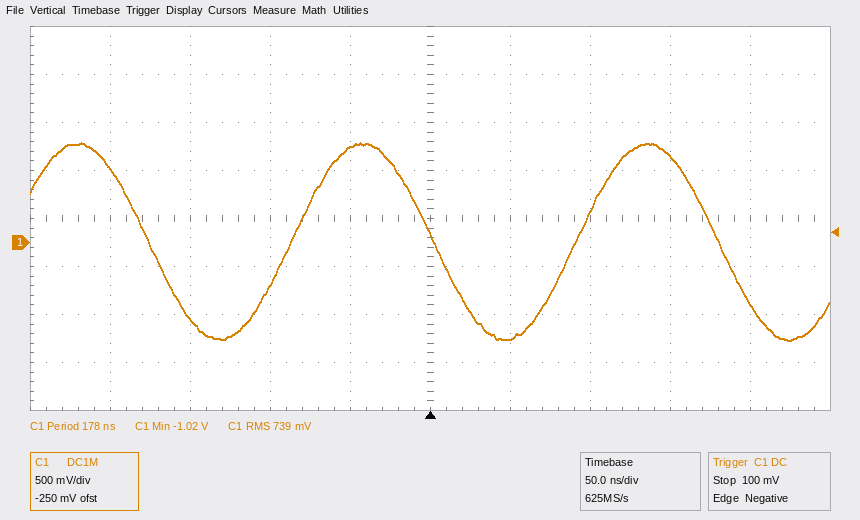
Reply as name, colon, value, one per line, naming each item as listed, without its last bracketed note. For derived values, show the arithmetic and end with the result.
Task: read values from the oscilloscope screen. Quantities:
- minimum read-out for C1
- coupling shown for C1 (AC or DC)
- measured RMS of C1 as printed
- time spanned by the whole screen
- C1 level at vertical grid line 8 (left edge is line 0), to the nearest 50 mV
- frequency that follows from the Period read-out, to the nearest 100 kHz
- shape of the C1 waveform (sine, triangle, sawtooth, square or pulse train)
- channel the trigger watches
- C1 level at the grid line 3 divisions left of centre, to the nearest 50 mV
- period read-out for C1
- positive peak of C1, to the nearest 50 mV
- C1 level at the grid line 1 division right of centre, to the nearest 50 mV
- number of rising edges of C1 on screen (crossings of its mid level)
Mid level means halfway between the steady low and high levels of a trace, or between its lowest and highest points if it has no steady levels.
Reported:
minimum read-out for C1: -1.02 V
coupling shown for C1: DC
measured RMS of C1 as printed: 739 mV
time spanned by the whole screen: 500 ns
C1 level at vertical grid line 8 (left edge is line 0), to the nearest 50 mV: 900 mV
frequency that follows from the Period read-out, to the nearest 100 kHz: 1 / 178 ns ≈ 5.6 MHz
shape of the C1 waveform: sine
channel the trigger watches: C1
C1 level at the grid line 3 divisions left of centre, to the nearest 50 mV: -800 mV
period read-out for C1: 178 ns
positive peak of C1, to the nearest 50 mV: 1.05 V
C1 level at the grid line 1 division right of centre, to the nearest 50 mV: -1.00 V
number of rising edges of C1 on screen: 2
